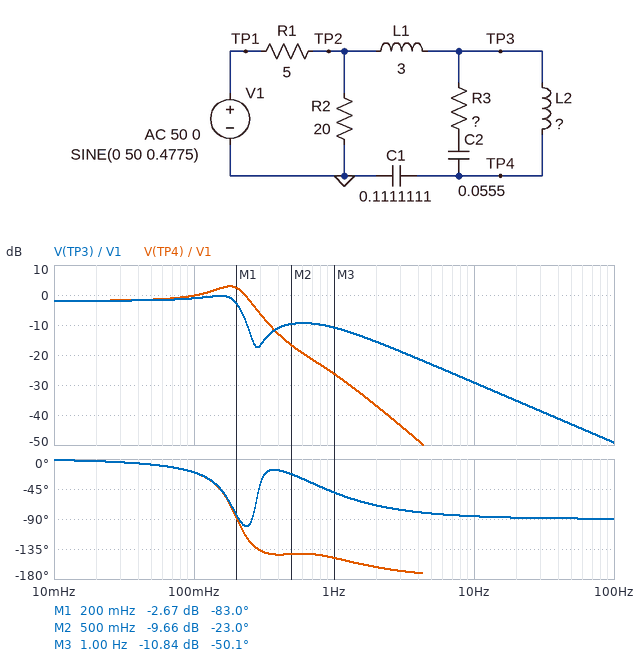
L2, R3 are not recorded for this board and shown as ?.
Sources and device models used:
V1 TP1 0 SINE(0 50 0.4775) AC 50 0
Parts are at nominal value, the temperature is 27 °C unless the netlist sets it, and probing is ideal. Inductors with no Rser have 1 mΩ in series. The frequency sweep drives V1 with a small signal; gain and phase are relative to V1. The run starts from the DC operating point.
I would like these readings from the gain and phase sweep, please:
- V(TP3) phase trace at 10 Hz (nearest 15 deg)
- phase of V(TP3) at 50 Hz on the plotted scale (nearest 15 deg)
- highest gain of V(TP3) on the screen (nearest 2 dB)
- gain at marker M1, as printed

-90 deg
-90 deg
0 dB
-2.67 dB
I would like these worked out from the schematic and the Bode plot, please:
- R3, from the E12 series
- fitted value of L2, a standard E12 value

8.2 Ω
2.2 H
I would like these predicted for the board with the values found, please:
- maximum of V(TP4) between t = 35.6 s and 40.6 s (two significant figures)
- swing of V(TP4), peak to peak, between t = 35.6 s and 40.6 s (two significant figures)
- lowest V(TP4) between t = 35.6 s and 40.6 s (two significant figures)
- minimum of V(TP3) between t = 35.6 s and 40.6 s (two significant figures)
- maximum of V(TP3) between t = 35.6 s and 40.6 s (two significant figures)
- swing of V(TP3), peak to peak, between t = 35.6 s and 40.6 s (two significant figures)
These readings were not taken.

7.8 V
16 V
-7.8 V
-16 V
16 V
32 V
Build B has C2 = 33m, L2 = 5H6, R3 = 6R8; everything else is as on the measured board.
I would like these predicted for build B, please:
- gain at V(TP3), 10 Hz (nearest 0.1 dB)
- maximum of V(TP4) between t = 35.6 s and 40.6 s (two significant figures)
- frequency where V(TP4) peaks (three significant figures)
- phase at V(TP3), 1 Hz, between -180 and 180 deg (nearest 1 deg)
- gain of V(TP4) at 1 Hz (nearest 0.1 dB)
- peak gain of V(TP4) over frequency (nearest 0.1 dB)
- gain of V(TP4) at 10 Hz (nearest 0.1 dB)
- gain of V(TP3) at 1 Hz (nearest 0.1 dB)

-30.7 dB
4.8 V
145 mHz
-78 deg
-24.3 dB
5.1 dB
-64.3 dB
-7.3 dB
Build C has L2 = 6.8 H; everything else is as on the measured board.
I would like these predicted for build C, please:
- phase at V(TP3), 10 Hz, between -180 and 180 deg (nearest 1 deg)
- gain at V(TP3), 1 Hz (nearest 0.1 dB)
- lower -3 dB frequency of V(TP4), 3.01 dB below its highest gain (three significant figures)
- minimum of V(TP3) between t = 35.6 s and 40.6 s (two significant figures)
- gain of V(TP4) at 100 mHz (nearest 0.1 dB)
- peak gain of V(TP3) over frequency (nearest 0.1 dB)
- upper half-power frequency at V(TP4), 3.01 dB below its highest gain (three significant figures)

-88 deg
-8.8 dB
94.8 mHz
-31 V
2.5 dB
-1.2 dB
152 mHz
